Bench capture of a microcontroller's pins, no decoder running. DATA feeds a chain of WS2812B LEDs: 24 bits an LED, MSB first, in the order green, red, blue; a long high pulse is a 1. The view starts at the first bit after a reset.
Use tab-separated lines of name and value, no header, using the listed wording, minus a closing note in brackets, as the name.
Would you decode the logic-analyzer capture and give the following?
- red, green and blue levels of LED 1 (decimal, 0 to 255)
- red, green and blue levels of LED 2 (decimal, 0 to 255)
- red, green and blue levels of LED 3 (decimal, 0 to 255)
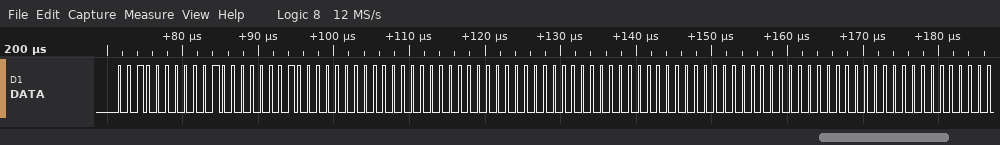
red, green and blue levels of LED 1	32, 32, 32
red, green and blue levels of LED 2	0, 0, 0
red, green and blue levels of LED 3	0, 0, 0
